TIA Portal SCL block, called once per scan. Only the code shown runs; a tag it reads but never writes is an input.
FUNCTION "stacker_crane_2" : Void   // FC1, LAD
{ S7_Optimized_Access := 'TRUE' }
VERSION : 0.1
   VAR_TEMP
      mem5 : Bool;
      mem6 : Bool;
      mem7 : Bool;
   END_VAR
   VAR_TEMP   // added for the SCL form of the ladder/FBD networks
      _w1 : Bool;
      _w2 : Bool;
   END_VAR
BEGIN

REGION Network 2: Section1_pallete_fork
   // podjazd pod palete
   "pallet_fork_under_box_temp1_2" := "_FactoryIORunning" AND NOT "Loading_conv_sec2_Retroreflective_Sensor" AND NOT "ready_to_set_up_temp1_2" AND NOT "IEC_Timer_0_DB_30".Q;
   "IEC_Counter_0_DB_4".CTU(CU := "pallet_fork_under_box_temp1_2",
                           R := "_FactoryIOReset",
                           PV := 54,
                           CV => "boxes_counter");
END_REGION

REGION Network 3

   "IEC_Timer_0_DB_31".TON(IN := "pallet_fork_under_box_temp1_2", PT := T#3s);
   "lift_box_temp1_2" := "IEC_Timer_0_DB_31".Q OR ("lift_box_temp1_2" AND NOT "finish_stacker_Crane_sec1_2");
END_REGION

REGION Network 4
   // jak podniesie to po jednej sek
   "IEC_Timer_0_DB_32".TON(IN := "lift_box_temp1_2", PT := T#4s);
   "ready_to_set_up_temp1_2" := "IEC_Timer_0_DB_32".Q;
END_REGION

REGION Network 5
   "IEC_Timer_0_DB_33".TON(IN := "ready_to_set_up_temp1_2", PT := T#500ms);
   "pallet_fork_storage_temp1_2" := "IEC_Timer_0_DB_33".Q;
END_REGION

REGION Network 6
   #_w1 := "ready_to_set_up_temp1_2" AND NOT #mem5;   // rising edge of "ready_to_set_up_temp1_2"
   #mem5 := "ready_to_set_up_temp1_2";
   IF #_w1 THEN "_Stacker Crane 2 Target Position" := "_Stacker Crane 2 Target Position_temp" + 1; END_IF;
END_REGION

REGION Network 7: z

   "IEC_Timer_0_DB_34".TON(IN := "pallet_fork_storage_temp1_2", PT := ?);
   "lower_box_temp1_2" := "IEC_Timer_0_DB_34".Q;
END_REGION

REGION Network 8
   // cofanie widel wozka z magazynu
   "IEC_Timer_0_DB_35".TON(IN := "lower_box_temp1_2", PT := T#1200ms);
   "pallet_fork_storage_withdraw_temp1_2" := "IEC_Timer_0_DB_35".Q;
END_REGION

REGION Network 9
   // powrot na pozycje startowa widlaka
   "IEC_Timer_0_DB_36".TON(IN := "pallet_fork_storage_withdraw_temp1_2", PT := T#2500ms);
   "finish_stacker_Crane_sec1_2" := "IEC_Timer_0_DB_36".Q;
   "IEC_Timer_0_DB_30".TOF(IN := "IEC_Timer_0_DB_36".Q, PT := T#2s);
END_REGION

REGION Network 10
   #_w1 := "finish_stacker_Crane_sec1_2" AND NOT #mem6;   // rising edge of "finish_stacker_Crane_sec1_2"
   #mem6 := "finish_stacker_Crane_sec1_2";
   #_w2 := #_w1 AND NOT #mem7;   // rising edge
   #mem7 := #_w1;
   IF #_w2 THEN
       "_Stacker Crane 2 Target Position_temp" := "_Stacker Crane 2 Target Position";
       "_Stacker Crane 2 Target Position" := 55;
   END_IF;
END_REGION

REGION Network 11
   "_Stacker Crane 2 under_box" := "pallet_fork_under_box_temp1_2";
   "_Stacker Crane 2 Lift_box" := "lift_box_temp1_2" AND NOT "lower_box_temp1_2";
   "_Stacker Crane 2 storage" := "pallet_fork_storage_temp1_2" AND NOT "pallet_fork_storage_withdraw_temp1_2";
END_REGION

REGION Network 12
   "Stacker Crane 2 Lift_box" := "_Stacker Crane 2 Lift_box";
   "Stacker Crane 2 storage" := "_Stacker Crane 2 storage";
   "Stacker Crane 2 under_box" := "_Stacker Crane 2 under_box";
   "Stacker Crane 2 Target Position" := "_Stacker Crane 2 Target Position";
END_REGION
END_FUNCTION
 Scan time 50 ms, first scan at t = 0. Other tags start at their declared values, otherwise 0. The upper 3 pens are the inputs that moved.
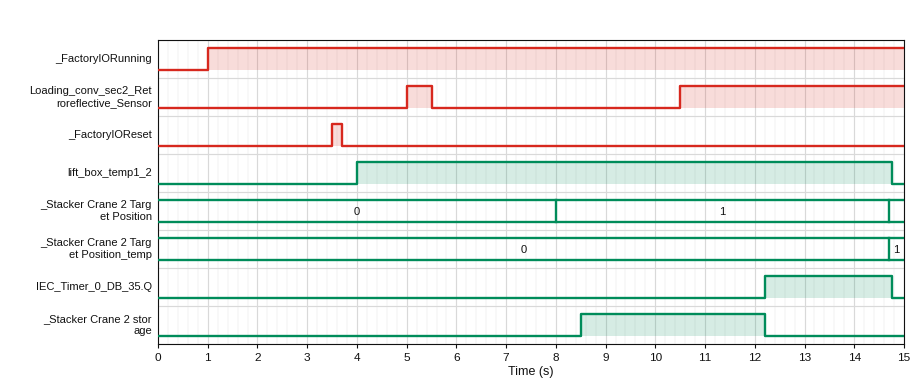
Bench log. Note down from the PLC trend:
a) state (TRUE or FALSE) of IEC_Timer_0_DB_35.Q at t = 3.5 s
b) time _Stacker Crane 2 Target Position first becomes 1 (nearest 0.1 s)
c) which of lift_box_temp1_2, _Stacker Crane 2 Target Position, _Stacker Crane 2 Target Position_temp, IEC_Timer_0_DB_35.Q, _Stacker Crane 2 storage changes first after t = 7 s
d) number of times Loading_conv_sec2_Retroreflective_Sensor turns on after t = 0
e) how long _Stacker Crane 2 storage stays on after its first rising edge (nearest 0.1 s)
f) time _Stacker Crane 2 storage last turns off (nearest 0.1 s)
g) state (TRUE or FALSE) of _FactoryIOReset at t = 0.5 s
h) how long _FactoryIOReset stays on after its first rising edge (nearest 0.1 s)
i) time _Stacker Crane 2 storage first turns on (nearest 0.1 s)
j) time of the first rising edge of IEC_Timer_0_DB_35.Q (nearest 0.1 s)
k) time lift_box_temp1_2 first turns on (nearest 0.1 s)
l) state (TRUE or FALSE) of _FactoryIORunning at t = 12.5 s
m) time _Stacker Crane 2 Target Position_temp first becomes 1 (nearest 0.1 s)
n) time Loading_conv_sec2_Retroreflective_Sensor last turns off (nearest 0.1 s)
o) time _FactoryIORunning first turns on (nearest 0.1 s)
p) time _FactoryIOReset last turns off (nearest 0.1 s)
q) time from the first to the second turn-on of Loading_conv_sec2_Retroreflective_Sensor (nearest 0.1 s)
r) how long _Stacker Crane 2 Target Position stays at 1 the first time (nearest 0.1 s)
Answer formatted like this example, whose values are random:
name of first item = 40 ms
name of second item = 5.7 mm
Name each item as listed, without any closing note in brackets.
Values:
state (TRUE or FALSE) of IEC_Timer_0_DB_35.Q at t = 3.5 s = FALSE
time _Stacker Crane 2 Target Position first becomes 1 = 8.0 s
which of lift_box_temp1_2, _Stacker Crane 2 Target Position, _Stacker Crane 2 Target Position_temp, IEC_Timer_0_DB_35.Q, _Stacker Crane 2 storage changes first after t = 7 s = _Stacker Crane 2 Target Position
number of times Loading_conv_sec2_Retroreflective_Sensor turns on after t = 0 = 2
how long _Stacker Crane 2 storage stays on after its first rising edge = 3.7 s
time _Stacker Crane 2 storage last turns off = 12.2 s
state (TRUE or FALSE) of _FactoryIOReset at t = 0.5 s = FALSE
how long _FactoryIOReset stays on after its first rising edge = 0.2 s
time _Stacker Crane 2 storage first turns on = 8.5 s
time of the first rising edge of IEC_Timer_0_DB_35.Q = 12.2 s
time lift_box_temp1_2 first turns on = 4.0 s
state (TRUE or FALSE) of _FactoryIORunning at t = 12.5 s = TRUE
time _Stacker Crane 2 Target Position_temp first becomes 1 = 14.7 s
time Loading_conv_sec2_Retroreflective_Sensor last turns off = 5.5 s
time _FactoryIORunning first turns on = 1.0 s
time _FactoryIOReset last turns off = 3.7 s
time from the first to the second turn-on of Loading_conv_sec2_Retroreflective_Sensor = 5.5 s
how long _Stacker Crane 2 Target Position stays at 1 the first time = 6.7 s
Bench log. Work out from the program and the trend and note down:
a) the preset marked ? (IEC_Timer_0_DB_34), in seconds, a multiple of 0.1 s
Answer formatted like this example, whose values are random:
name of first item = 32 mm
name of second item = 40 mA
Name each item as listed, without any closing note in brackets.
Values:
the preset marked ? (IEC_Timer_0_DB_34), in seconds, a multiple of 0.1 s = 2.5 s
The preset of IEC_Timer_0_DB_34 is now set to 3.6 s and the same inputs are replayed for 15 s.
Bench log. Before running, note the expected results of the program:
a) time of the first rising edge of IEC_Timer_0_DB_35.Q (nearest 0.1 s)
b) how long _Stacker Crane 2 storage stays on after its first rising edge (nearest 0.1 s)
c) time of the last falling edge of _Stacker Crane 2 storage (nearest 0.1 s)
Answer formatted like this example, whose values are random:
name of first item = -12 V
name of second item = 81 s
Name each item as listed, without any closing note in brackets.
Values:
time of the first rising edge of IEC_Timer_0_DB_35.Q = 13.3 s
how long _Stacker Crane 2 storage stays on after its first rising edge = 4.8 s
time of the last falling edge of _Stacker Crane 2 storage = 13.3 s
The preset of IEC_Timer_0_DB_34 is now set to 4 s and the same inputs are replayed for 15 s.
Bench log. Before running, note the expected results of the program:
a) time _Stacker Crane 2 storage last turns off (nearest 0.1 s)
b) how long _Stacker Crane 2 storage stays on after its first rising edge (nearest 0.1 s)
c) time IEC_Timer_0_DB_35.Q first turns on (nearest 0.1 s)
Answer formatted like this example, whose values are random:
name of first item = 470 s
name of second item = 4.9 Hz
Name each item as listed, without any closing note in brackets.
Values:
time _Stacker Crane 2 storage last turns off = 13.7 s
how long _Stacker Crane 2 storage stays on after its first rising edge = 5.2 s
time IEC_Timer_0_DB_35.Q first turns on = 13.7 s
